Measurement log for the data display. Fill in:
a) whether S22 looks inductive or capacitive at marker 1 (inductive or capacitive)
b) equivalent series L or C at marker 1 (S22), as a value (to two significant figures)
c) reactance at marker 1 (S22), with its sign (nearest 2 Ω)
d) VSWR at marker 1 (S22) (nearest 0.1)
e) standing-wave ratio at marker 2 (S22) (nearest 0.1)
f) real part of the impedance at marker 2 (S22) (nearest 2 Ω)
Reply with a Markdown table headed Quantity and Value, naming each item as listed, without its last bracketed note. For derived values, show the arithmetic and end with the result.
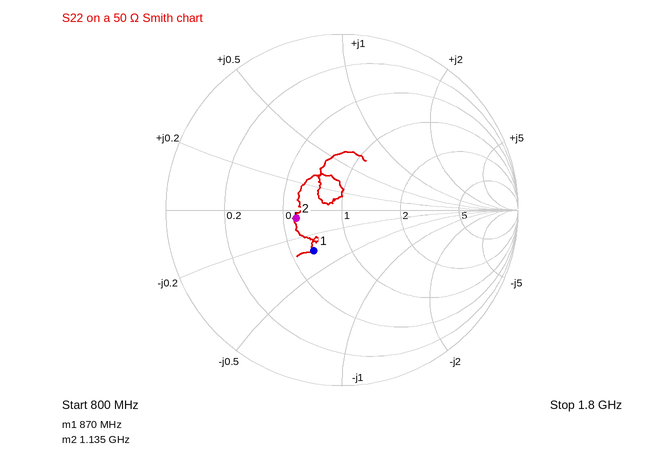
| Quantity | Value |
|---|---|
| whether S22 looks inductive or capacitive at marker 1 | capacitive |
| equivalent series L or C at marker 1 (S22), as a value | C = 1/(2π × 870 MHz × 16 Ω) ≈ 11 pF |
| reactance at marker 1 (S22), with its sign | -16 Ω |
| VSWR at marker 1 (S22) | 1.8 |
| standing-wave ratio at marker 2 (S22) | 1.7 |
| real part of the impedance at marker 2 (S22) | 30 Ω |
